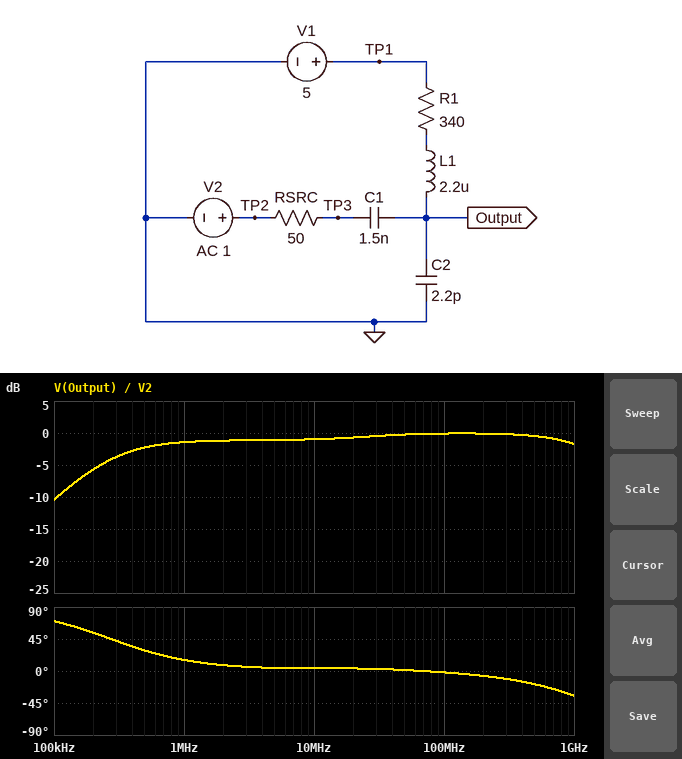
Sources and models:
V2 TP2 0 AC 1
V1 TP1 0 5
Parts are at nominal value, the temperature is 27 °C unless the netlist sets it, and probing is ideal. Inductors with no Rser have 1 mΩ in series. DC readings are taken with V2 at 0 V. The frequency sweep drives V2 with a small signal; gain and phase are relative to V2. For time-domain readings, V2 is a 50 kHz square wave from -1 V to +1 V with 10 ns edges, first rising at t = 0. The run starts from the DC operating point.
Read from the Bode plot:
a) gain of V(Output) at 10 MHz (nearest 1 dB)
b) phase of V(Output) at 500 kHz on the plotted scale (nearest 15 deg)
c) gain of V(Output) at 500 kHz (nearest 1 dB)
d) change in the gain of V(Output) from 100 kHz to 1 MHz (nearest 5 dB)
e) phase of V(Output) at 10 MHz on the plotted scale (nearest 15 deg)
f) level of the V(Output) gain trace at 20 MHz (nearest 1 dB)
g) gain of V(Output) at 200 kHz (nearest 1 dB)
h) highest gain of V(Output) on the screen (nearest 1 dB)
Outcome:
-1 dB
30 deg
-2 dB
10 dB
0 deg
-1 dB
-6 dB
0 dB
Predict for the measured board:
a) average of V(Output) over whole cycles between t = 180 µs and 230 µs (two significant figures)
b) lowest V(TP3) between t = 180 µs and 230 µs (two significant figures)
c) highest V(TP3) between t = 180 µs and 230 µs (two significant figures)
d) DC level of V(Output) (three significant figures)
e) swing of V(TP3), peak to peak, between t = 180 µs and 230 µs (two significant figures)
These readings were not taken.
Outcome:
5.0 V
-1.0 V
1.0 V
5.00 V
2.0 V
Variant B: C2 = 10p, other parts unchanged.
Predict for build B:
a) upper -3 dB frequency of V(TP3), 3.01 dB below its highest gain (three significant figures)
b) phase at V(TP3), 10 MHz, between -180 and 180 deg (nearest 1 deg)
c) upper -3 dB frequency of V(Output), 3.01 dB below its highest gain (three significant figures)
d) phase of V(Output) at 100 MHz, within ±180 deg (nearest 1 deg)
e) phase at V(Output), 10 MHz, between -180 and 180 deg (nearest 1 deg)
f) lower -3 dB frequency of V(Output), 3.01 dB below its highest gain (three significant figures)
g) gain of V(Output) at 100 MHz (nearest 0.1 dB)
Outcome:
324 MHz
1 deg
341 MHz
-15 deg
2 deg
341 kHz
-0.4 dB
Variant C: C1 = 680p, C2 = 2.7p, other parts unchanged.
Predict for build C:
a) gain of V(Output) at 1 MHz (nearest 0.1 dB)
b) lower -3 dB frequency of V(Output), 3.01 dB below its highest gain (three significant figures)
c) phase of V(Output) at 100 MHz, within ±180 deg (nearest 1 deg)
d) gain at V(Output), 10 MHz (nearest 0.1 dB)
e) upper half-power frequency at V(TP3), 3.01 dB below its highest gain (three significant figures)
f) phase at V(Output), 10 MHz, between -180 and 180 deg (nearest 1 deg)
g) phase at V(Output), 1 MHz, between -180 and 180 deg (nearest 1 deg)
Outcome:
-2.4 dB
780 kHz
-3 deg
-0.9 dB
1.19 GHz
5 deg
32 deg
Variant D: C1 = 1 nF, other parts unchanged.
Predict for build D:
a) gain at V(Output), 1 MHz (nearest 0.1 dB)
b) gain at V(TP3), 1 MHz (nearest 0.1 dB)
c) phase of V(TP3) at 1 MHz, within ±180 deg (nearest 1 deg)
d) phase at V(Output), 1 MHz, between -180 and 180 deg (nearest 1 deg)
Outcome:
-1.8 dB
-1.0 dB
-3 deg
23 deg
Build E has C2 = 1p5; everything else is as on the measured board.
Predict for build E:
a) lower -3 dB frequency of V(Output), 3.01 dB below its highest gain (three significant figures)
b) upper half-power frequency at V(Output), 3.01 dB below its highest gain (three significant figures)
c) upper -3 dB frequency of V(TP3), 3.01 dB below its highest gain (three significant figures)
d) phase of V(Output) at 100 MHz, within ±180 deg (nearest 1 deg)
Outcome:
365 kHz
2.15 GHz
2.13 GHz
-1 deg
